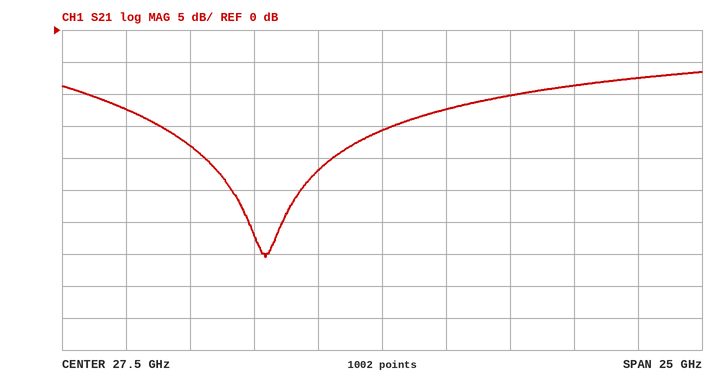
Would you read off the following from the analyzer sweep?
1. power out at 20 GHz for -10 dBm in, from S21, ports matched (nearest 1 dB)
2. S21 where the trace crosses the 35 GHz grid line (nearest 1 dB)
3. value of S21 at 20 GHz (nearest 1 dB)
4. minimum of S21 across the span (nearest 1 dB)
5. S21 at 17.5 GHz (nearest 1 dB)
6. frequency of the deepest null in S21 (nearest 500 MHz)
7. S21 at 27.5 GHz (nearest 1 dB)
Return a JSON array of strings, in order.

["-28 dBm", "-9 dB", "-18 dB", "-35 dB", "-12 dB", "23.0 GHz", "-16 dB"]
